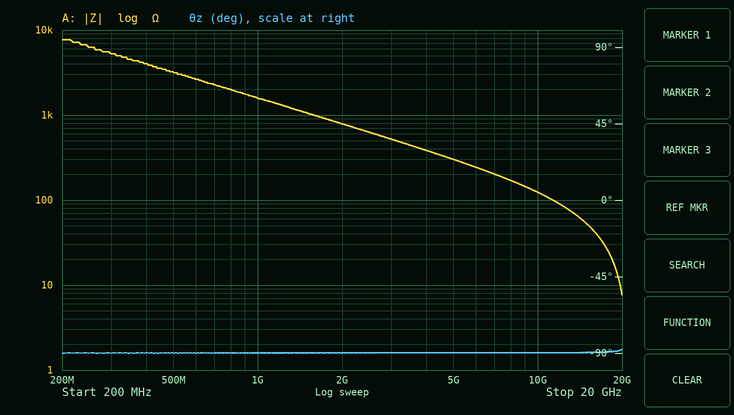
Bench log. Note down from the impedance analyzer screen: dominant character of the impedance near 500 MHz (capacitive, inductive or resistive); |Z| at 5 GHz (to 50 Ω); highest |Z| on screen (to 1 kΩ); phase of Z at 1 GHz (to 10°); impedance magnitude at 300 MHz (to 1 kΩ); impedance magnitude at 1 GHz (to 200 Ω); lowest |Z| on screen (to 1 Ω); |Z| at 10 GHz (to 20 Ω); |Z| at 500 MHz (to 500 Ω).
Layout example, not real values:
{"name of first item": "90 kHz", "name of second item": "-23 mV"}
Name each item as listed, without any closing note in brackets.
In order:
{"dominant character of the impedance near 500 MHz": "capacitive", "|Z| at 5 GHz": "300 Ω", "highest |Z| on screen": "8 kΩ", "phase of Z at 1 GHz": "-90°", "impedance magnitude at 300 MHz": "5 kΩ", "impedance magnitude at 1 GHz": "1.6 kΩ", "lowest |Z| on screen": "8 Ω", "|Z| at 10 GHz": "120 Ω", "|Z| at 500 MHz": "3.0 kΩ"}
